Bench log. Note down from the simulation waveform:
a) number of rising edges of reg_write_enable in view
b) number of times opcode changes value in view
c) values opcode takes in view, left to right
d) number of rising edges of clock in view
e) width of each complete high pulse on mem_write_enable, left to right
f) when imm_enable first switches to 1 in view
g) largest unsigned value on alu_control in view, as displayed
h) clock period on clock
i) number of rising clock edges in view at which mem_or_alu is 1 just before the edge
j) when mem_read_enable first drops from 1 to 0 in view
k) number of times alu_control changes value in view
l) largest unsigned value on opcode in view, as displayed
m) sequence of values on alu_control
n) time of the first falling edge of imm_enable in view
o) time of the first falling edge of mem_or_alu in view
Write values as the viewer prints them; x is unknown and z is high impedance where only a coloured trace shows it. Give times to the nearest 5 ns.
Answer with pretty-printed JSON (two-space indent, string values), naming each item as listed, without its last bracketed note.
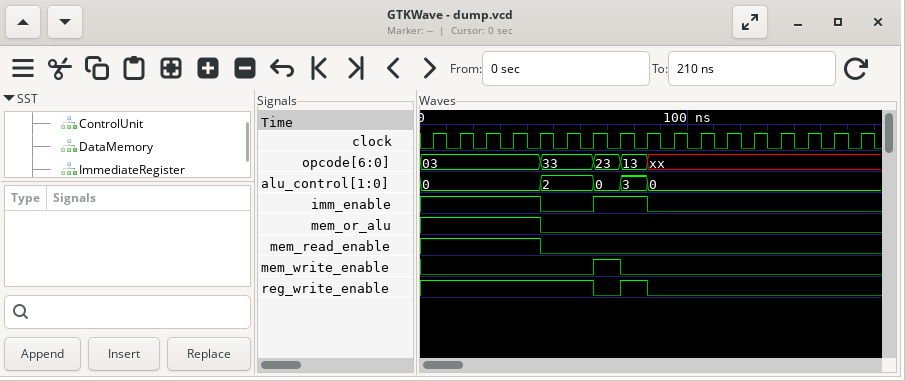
{
  "number of rising edges of reg_write_enable in view": "1",
  "number of times opcode changes value in view": "4",
  "values opcode takes in view, left to right": "03, 33, 23, 13, xx",
  "number of rising edges of clock in view": "17",
  "width of each complete high pulse on mem_write_enable, left to right": "10 ns",
  "when imm_enable first switches to 1 in view": "65 ns",
  "largest unsigned value on alu_control in view, as displayed": "3",
  "clock period on clock": "10 ns",
  "number of rising clock edges in view at which mem_or_alu is 1 just before the edge": "5",
  "when mem_read_enable first drops from 1 to 0 in view": "45 ns",
  "number of times alu_control changes value in view": "4",
  "largest unsigned value on opcode in view, as displayed": "33",
  "sequence of values on alu_control": "0, 2, 0, 3, 0",
  "time of the first falling edge of imm_enable in view": "45 ns",
  "time of the first falling edge of mem_or_alu in view": "45 ns"
}
